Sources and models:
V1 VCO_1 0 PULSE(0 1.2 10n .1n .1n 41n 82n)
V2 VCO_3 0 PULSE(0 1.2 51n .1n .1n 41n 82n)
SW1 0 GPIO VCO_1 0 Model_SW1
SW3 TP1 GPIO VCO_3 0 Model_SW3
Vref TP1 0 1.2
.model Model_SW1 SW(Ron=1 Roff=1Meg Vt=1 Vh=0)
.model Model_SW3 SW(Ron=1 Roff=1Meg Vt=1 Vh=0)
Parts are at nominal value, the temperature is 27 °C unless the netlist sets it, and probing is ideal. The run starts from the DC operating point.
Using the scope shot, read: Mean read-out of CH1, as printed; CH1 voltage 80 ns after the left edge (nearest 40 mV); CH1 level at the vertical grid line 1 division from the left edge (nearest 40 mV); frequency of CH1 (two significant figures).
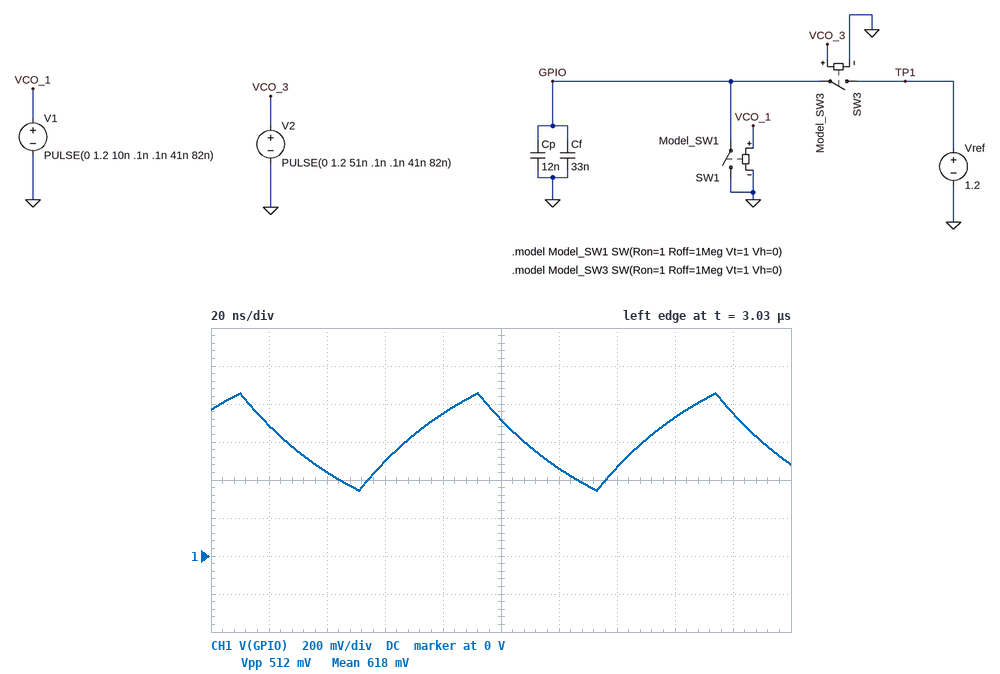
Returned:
618 mV
760 mV
680 mV
12 MHz
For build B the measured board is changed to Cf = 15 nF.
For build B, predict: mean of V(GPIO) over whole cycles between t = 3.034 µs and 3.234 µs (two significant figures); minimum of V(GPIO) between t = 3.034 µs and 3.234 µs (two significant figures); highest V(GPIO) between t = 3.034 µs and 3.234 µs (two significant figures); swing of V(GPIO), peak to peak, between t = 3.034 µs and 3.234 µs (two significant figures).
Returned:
600 mV
220 mV
980 mV
770 mV
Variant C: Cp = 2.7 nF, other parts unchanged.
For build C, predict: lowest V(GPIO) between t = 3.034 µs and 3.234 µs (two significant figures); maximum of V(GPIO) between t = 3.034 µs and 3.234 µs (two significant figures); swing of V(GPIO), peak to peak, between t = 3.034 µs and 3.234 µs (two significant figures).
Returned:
290 mV
910 mV
620 mV
